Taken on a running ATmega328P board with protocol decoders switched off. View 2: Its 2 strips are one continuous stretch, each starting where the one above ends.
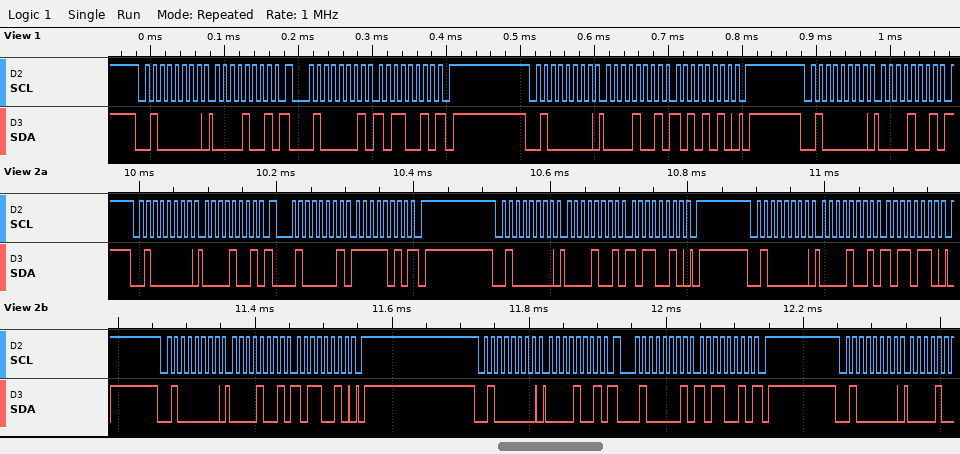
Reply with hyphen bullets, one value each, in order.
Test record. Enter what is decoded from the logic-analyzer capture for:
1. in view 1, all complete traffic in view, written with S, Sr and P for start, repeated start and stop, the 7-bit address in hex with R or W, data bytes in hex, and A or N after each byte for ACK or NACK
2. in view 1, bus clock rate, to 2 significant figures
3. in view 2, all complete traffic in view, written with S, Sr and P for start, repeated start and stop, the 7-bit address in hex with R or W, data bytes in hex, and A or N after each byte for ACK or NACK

- S 20W A 09 A Sr 20R A B2 N P S 20W A 09 A AA A P S 20W A 09 A
- 100 kHz
- S 20W A 09 A Sr 20R A FA N P S 20W A 09 A B2 A P S 20W A 09 A B6 A P S 20W A 09 A B2 A P S 20W A 09 A Sr 20R A B2 N P S 20W A
